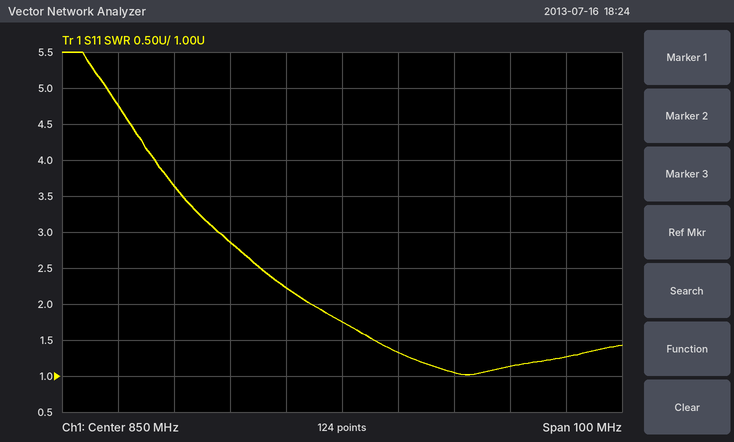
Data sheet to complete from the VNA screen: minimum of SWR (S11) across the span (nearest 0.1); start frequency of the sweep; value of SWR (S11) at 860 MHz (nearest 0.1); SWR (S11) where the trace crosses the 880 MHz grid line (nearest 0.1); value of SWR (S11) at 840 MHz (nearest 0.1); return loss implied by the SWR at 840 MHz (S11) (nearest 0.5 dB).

1.0
800 MHz
1.3
1.1
2.2
8.5 dB
